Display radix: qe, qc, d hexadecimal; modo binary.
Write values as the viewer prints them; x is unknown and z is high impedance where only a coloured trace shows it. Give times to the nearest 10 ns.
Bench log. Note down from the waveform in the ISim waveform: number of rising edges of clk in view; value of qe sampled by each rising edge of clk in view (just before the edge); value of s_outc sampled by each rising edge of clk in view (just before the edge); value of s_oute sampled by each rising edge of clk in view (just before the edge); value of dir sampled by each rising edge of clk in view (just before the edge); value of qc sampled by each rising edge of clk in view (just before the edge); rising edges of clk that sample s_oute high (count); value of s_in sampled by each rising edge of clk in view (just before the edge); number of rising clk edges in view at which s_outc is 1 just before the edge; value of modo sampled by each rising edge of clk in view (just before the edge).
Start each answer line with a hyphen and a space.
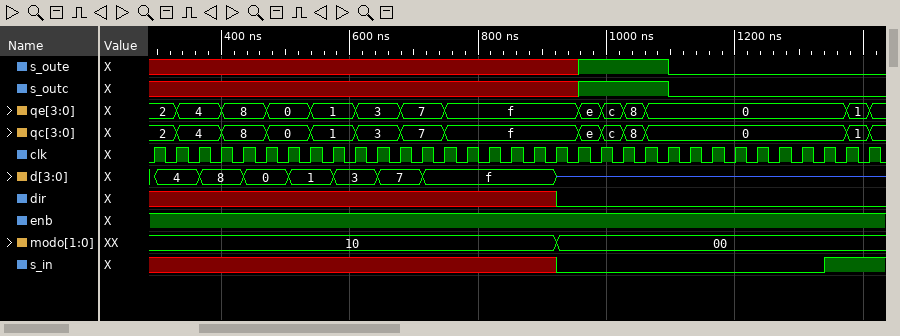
- 33
- 2, 2, 4, 4, 8, 8, 0, 0, 1, 1, 3, 3, 7, 7, f, f, f, f, f, f, e, c, 8, 0, 0, 0, 0, 0, 0, 0, 0, 0, 1
- x x x x x x x x x x x x x x x x x x x x 1 1 1 1 0 0 0 0 0 0 0 0 0
- x x x x x x x x x x x x x x x x x x x x 1 1 1 1 0 0 0 0 0 0 0 0 0
- x x x x x x x x x x x x x x x x x x x 0 0 0 0 0 0 0 0 0 0 0 0 0 0
- 2, 2, 4, 4, 8, 8, 0, 0, 1, 1, 3, 3, 7, 7, f, f, f, f, f, f, e, c, 8, 0, 0, 0, 0, 0, 0, 0, 0, 0, 1
- 4
- x x x x x x x x x x x x x x x x x x x 0 0 0 0 0 0 0 0 0 0 0 0 1 1
- 4
- 10, 10, 10, 10, 10, 10, 10, 10, 10, 10, 10, 10, 10, 10, 10, 10, 10, 10, 10, 00, 00, 00, 00, 00, 00, 00, 00, 00, 00, 00, 00, 00, 00
